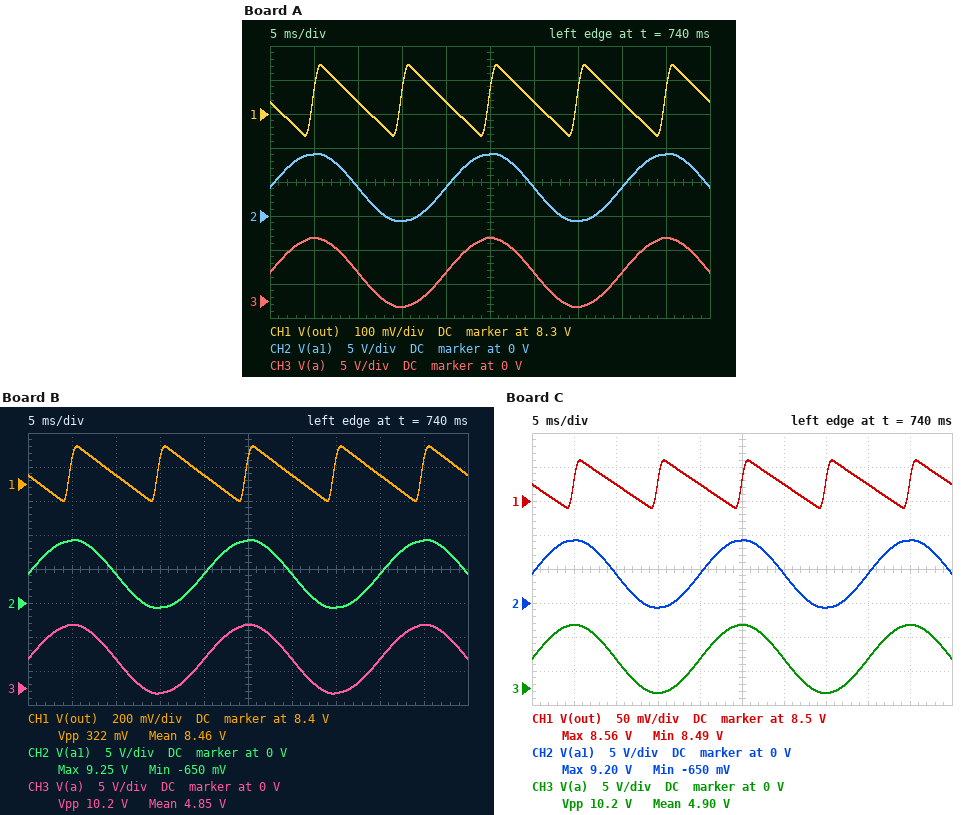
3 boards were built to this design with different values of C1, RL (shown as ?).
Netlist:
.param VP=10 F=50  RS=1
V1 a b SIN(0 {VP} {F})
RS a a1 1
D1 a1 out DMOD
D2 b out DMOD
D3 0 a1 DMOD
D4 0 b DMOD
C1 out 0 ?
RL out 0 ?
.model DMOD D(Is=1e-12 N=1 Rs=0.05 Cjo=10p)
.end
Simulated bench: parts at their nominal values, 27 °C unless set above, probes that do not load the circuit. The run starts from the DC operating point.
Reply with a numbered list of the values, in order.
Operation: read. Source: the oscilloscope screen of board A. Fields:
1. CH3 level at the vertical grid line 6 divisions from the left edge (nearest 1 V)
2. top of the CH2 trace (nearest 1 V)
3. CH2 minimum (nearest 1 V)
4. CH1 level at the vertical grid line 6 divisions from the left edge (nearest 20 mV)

1. 4 V
2. 9 V
3. -1 V
4. 8.34 V
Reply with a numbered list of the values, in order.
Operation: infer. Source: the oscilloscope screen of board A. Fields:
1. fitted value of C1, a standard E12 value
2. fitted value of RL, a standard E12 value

1. 1.2 mF
2. 270 Ω
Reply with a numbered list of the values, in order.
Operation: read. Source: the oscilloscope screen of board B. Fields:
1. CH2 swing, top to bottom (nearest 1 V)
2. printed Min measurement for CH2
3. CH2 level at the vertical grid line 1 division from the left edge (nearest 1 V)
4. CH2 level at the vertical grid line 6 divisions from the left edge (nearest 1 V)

1. 10 V
2. -650 mV
3. 9 V
4. 4 V
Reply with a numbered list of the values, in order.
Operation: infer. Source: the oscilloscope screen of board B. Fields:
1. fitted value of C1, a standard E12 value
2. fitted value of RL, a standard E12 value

1. 390 µF
2. 560 Ω
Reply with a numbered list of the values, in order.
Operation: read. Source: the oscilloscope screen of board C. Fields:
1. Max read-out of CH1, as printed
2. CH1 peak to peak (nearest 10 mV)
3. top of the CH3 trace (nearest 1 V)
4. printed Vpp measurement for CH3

1. 8.56 V
2. 70 mV
3. 9 V
4. 10.2 V
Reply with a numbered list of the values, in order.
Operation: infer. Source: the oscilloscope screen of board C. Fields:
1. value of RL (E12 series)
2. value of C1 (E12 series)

1. 680 Ω
2. 1.5 mF
